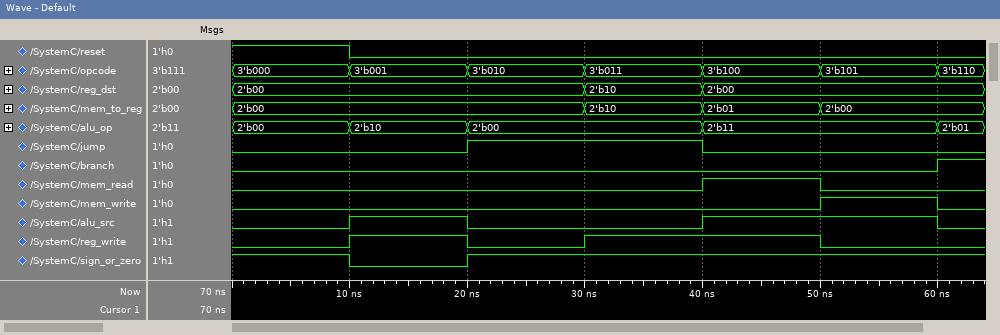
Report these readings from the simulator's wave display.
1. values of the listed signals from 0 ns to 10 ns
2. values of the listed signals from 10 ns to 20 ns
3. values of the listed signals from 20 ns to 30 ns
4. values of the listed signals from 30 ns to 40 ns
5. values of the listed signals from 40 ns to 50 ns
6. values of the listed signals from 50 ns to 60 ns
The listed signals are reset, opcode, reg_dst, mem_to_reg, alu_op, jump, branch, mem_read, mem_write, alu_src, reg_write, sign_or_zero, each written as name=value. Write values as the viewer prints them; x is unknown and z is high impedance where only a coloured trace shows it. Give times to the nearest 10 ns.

reset=1, opcode=3'b000, reg_dst=2'b00, mem_to_reg=2'b00, alu_op=2'b00, jump=0, branch=0, mem_read=0, mem_write=0, alu_src=0, reg_write=0, sign_or_zero=1
reset=0, opcode=3'b001, reg_dst=2'b00, mem_to_reg=2'b00, alu_op=2'b10, jump=0, branch=0, mem_read=0, mem_write=0, alu_src=1, reg_write=1, sign_or_zero=0
reset=0, opcode=3'b010, reg_dst=2'b00, mem_to_reg=2'b00, alu_op=2'b00, jump=1, branch=0, mem_read=0, mem_write=0, alu_src=0, reg_write=0, sign_or_zero=1
reset=0, opcode=3'b011, reg_dst=2'b10, mem_to_reg=2'b10, alu_op=2'b00, jump=1, branch=0, mem_read=0, mem_write=0, alu_src=0, reg_write=1, sign_or_zero=1
reset=0, opcode=3'b100, reg_dst=2'b00, mem_to_reg=2'b01, alu_op=2'b11, jump=0, branch=0, mem_read=1, mem_write=0, alu_src=1, reg_write=1, sign_or_zero=1
reset=0, opcode=3'b101, reg_dst=2'b00, mem_to_reg=2'b00, alu_op=2'b11, jump=0, branch=0, mem_read=0, mem_write=1, alu_src=1, reg_write=0, sign_or_zero=1
